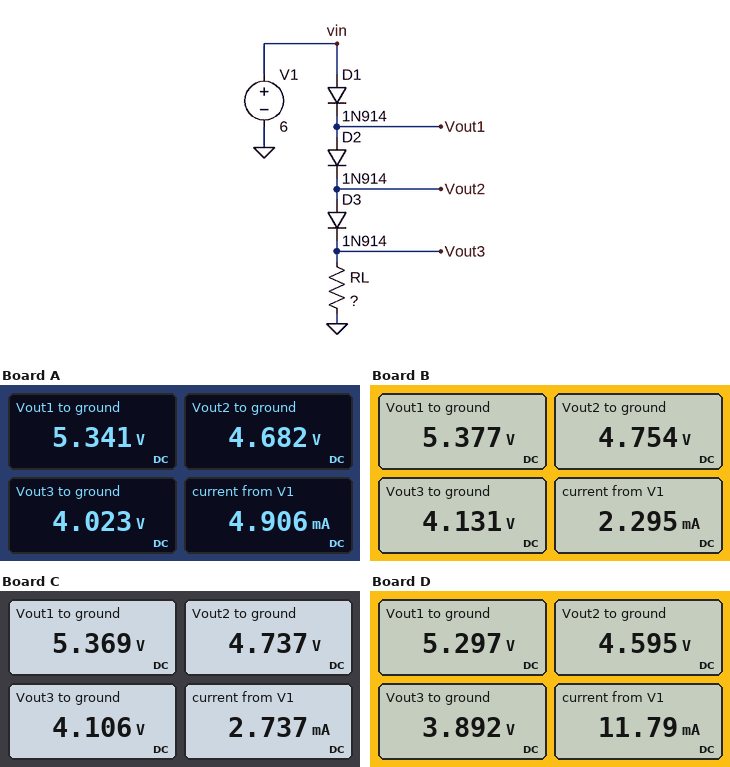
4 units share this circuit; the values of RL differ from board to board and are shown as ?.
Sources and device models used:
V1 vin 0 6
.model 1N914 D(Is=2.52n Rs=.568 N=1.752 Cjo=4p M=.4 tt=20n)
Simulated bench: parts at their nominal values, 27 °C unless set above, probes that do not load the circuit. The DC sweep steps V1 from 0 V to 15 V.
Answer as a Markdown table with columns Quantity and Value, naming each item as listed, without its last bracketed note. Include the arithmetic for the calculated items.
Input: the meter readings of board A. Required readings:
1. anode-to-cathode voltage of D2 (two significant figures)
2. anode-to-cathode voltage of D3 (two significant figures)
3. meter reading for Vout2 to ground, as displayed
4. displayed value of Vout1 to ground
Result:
| Quantity | Value |
|---|---|
| anode-to-cathode voltage of D2 | 5.341 V - 4.682 V = 660 mV |
| anode-to-cathode voltage of D3 | 4.682 V - 4.023 V = 660 mV |
| meter reading for Vout2 to ground, as displayed | 4.682 V |
| displayed value of Vout1 to ground | 5.341 V |
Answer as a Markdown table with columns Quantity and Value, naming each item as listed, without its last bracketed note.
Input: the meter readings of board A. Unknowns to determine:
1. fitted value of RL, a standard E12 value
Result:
| Quantity | Value |
|---|---|
| fitted value of RL, a standard E12 value | 820 Ω |
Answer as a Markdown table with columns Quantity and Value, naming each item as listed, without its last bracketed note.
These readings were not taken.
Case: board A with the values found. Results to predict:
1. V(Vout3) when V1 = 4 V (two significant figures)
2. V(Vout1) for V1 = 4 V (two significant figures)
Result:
| Quantity | Value |
|---|---|
| V(Vout3) when V1 = 4 V | 2.1 V |
| V(Vout1) for V1 = 4 V | 3.4 V |
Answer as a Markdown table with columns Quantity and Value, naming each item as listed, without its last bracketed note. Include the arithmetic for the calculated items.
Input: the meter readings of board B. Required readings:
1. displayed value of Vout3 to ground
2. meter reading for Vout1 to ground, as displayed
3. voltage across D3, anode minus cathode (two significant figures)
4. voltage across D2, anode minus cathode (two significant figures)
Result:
| Quantity | Value |
|---|---|
| displayed value of Vout3 to ground | 4.131 V |
| meter reading for Vout1 to ground, as displayed | 5.377 V |
| voltage across D3, anode minus cathode | 4.754 V - 4.131 V = 620 mV |
| voltage across D2, anode minus cathode | 5.377 V - 4.754 V = 620 mV |
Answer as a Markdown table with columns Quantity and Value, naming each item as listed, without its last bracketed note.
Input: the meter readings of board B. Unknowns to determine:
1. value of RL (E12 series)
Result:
| Quantity | Value |
|---|---|
| value of RL | 1.8 kΩ |
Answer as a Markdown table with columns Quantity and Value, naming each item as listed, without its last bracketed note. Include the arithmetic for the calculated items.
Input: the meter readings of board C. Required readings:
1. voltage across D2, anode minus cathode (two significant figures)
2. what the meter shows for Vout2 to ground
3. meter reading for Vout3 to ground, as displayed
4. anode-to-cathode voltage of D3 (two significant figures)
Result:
| Quantity | Value |
|---|---|
| voltage across D2, anode minus cathode | 5.369 V - 4.737 V = 630 mV |
| what the meter shows for Vout2 to ground | 4.737 V |
| meter reading for Vout3 to ground, as displayed | 4.106 V |
| anode-to-cathode voltage of D3 | 4.737 V - 4.106 V = 630 mV |
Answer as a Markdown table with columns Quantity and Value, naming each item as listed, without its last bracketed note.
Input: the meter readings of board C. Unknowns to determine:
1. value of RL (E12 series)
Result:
| Quantity | Value |
|---|---|
| value of RL | 1.5 kΩ |
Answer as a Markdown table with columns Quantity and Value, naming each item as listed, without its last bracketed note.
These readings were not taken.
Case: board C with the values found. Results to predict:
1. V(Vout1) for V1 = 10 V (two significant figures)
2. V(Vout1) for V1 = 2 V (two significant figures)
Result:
| Quantity | Value |
|---|---|
| V(Vout1) for V1 = 10 V | 9.3 V |
| V(Vout1) for V1 = 2 V | 1.5 V |
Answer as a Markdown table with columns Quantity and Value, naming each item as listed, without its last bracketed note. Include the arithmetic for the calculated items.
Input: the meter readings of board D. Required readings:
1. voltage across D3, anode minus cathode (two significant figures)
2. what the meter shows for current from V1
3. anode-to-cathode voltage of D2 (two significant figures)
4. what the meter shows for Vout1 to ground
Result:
| Quantity | Value |
|---|---|
| voltage across D3, anode minus cathode | 4.595 V - 3.892 V = 700 mV |
| what the meter shows for current from V1 | 11.79 mA |
| anode-to-cathode voltage of D2 | 5.297 V - 4.595 V = 700 mV |
| what the meter shows for Vout1 to ground | 5.297 V |
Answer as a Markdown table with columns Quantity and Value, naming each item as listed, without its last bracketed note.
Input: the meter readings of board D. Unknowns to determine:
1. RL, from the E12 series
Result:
| Quantity | Value |
|---|---|
| RL, from the E12 series | 330 Ω |
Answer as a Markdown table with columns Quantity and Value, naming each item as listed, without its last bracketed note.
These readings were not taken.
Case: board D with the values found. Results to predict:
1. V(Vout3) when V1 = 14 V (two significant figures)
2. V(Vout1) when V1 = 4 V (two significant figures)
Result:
| Quantity | Value |
|---|---|
| V(Vout3) when V1 = 14 V | 12 V |
| V(Vout1) when V1 = 4 V | 3.3 V |
